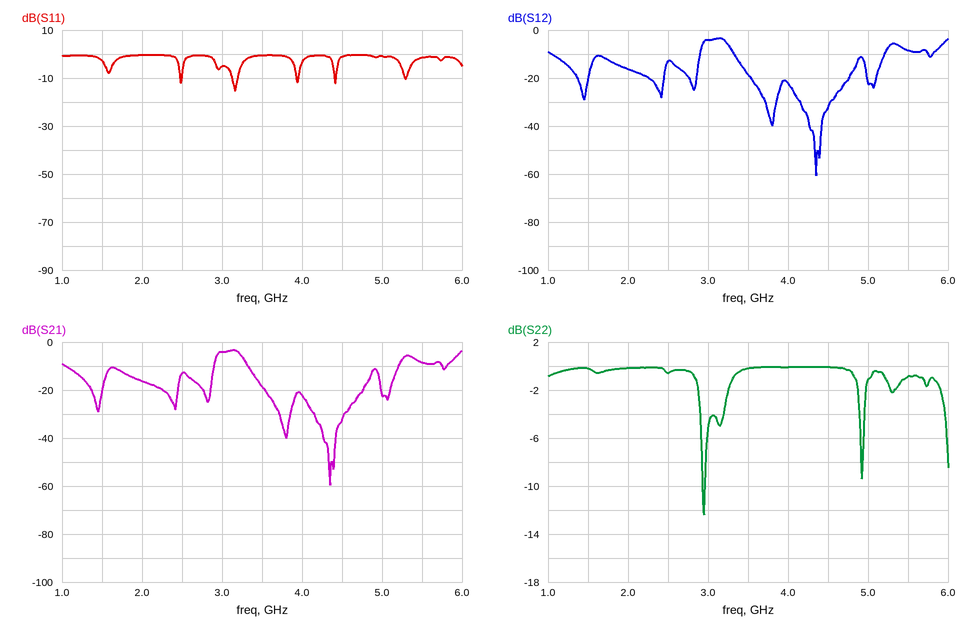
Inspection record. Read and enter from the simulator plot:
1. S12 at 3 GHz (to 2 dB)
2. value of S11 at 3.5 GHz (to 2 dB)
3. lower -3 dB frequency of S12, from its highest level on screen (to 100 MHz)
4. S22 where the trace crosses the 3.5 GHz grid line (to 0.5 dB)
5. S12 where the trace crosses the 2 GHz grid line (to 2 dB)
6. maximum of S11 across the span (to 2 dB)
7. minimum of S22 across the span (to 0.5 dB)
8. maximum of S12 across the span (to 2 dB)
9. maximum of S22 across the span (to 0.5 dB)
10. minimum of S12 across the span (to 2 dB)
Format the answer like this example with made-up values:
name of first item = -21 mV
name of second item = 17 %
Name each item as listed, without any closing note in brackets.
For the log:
S12 at 3 GHz = -4 dB
value of S11 at 3.5 GHz = 0 dB
lower -3 dB frequency of S12, from its highest level on screen = 2.9 GHz
S22 where the trace crosses the 3.5 GHz grid line = 0.0 dB
S12 where the trace crosses the 2 GHz grid line = -16 dB
maximum of S11 across the span = 0 dB
minimum of S22 across the span = -12.5 dB
maximum of S12 across the span = -4 dB
maximum of S22 across the span = 0.0 dB
minimum of S12 across the span = -60 dB
